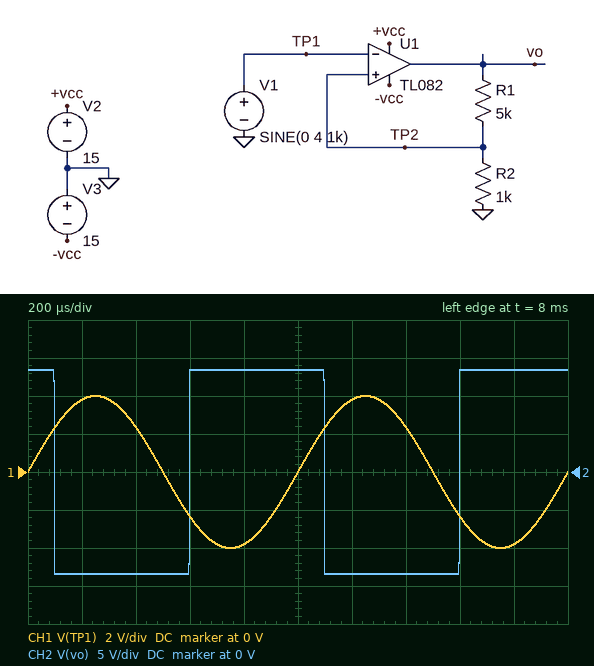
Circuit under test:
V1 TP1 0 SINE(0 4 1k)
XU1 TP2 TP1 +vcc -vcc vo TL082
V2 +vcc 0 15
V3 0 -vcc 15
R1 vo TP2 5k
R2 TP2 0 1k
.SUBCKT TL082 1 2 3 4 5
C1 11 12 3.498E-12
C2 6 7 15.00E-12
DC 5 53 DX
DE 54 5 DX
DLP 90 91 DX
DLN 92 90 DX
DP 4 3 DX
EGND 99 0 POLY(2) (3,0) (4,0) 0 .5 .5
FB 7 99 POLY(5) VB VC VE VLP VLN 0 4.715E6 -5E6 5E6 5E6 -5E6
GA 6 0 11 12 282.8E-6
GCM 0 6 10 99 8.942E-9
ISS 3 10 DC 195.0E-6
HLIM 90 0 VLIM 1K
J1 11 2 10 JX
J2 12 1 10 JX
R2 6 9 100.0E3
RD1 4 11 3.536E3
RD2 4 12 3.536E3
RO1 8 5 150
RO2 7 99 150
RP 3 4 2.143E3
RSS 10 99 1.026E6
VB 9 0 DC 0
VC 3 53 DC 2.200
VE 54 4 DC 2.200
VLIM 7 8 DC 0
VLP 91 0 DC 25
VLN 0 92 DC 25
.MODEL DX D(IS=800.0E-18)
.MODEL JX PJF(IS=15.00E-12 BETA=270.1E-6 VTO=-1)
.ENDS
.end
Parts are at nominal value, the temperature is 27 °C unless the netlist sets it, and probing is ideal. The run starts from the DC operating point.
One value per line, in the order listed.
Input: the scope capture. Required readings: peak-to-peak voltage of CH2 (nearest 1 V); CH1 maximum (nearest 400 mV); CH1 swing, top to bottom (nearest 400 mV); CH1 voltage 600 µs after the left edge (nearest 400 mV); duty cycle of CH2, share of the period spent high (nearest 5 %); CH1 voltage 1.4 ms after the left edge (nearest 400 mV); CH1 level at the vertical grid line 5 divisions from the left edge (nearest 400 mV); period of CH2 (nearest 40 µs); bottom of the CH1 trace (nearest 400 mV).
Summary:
27 V
4.0 V
8.0 V
-2.4 V
50 %
2.4 V
0 V
1.00 ms
-4.0 V
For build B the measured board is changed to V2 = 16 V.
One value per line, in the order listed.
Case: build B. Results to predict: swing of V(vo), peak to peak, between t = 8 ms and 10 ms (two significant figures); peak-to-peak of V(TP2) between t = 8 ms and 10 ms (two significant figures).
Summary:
28 V
4.7 V
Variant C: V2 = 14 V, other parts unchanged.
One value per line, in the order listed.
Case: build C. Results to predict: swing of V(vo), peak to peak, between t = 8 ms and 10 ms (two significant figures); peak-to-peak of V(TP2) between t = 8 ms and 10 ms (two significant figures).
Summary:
26 V
4.3 V
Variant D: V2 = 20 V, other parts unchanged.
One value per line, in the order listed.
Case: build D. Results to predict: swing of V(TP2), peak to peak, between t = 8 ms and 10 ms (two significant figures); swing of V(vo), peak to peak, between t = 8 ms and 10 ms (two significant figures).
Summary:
5.3 V
32 V
